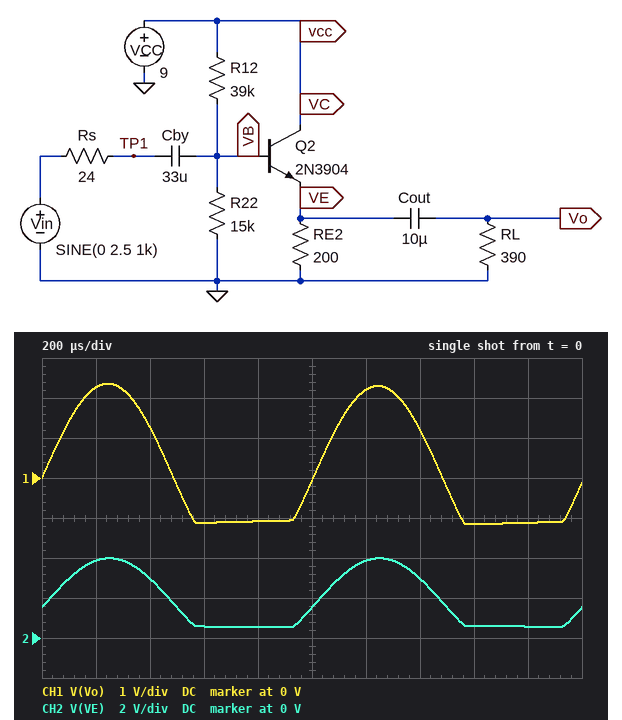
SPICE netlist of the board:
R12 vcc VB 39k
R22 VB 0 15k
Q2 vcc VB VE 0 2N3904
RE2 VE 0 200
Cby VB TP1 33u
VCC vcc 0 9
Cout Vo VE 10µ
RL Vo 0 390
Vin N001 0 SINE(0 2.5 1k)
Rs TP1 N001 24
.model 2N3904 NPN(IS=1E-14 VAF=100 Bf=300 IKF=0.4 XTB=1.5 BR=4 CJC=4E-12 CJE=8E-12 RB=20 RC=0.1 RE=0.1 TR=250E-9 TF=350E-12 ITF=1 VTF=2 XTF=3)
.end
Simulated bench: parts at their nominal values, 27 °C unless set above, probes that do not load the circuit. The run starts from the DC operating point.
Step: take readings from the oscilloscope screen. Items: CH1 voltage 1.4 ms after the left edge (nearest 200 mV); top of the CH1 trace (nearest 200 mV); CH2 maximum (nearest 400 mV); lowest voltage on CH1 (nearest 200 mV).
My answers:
1.2 V
2.4 V
4.0 V
-1.2 V
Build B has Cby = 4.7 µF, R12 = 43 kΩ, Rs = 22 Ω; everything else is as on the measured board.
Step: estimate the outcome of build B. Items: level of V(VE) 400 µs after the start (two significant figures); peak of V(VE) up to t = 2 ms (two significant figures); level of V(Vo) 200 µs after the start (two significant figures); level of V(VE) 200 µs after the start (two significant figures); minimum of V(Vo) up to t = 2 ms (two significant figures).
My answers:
2.8 V
3.8 V
2.3 V
3.7 V
-1.1 V
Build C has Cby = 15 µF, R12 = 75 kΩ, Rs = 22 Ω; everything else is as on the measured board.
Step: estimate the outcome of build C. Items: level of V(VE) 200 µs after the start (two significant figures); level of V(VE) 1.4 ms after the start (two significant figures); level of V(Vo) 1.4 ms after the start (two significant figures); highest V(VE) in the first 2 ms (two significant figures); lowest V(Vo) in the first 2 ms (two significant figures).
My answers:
3.0 V
2.1 V
1.1 V
3.1 V
-640 mV
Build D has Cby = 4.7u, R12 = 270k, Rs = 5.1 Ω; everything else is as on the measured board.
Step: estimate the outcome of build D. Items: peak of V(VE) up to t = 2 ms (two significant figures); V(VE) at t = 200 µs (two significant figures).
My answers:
2.2 V
2.1 V
